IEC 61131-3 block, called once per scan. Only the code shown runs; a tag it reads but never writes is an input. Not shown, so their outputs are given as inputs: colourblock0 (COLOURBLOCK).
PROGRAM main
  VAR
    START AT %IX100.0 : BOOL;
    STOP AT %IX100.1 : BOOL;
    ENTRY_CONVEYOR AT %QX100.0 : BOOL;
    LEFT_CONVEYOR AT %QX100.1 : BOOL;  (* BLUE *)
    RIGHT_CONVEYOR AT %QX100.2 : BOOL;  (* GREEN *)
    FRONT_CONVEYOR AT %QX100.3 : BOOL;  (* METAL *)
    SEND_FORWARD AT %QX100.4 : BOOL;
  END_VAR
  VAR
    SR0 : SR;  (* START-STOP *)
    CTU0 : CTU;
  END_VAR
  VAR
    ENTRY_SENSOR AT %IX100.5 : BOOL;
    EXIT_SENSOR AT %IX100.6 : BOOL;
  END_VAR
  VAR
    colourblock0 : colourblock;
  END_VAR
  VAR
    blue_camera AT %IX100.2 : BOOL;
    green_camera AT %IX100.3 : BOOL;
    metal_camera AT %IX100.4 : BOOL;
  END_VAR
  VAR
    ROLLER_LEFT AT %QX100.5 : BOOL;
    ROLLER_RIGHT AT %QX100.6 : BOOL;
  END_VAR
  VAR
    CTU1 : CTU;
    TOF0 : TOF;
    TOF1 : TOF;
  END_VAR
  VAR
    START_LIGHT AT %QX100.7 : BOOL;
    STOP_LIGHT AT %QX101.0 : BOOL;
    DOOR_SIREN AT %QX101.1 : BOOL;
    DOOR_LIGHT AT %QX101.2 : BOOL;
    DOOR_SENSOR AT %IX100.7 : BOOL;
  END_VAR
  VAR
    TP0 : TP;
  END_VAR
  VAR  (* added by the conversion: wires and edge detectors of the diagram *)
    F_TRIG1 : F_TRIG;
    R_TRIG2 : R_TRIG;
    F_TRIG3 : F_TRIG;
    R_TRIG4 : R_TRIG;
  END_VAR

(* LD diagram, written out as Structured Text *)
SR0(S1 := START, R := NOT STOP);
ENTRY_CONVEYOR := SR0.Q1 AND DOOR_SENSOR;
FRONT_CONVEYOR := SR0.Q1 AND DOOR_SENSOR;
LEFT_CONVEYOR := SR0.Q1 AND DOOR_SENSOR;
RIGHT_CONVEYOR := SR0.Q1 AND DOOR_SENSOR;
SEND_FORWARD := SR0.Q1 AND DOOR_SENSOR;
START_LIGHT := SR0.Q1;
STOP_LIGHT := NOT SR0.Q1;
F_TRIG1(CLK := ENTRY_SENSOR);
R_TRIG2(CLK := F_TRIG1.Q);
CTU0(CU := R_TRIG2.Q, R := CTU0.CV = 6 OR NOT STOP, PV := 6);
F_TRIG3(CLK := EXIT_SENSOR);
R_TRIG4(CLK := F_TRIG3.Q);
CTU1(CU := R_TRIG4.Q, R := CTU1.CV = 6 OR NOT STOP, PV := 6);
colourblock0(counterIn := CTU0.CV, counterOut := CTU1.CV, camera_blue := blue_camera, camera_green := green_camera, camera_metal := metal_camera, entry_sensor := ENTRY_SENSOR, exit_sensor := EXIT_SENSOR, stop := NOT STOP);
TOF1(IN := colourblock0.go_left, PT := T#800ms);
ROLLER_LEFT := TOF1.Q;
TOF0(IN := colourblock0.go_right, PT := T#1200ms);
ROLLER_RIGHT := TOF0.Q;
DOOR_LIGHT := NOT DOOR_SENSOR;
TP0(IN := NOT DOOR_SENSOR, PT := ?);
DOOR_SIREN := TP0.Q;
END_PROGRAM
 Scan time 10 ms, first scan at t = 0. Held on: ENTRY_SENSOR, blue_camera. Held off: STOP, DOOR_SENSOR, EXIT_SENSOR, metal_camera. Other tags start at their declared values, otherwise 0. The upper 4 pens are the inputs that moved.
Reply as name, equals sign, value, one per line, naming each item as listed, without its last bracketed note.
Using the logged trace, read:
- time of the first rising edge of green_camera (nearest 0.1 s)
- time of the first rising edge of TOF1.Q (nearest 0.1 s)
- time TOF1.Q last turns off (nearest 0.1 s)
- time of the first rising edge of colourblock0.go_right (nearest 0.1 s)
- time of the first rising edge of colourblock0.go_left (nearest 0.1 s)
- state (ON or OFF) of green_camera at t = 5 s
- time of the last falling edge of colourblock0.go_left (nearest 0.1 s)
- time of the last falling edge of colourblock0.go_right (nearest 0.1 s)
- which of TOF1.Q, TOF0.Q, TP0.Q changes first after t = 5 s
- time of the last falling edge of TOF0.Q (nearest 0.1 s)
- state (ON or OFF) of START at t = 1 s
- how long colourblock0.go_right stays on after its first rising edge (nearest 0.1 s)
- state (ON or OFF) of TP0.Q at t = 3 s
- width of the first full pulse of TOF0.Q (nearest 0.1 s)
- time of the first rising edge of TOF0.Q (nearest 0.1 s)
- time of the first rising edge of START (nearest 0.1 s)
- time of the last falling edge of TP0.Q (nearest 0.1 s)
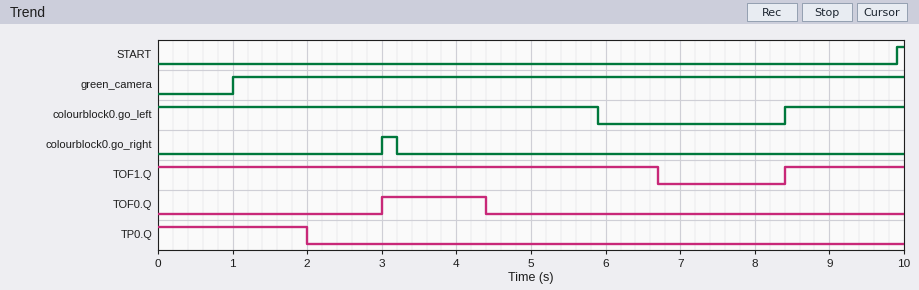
time of the first rising edge of green_camera = 1.0 s
time of the first rising edge of TOF1.Q = 8.4 s
time TOF1.Q last turns off = 6.7 s
time of the first rising edge of colourblock0.go_right = 3.0 s
time of the first rising edge of colourblock0.go_left = 8.4 s
state (ON or OFF) of green_camera at t = 5 s = ON
time of the last falling edge of colourblock0.go_left = 5.9 s
time of the last falling edge of colourblock0.go_right = 3.2 s
which of TOF1.Q, TOF0.Q, TP0.Q changes first after t = 5 s = TOF1.Q
time of the last falling edge of TOF0.Q = 4.4 s
state (ON or OFF) of START at t = 1 s = OFF
how long colourblock0.go_right stays on after its first rising edge = 0.2 s
state (ON or OFF) of TP0.Q at t = 3 s = OFF
width of the first full pulse of TOF0.Q = 1.4 s
time of the first rising edge of TOF0.Q = 3.0 s
time of the first rising edge of START = 9.9 s
time of the last falling edge of TP0.Q = 2.0 s
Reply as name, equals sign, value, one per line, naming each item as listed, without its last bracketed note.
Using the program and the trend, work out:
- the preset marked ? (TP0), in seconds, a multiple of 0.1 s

the preset marked ? (TP0), in seconds, a multiple of 0.1 s = 2.0 s
